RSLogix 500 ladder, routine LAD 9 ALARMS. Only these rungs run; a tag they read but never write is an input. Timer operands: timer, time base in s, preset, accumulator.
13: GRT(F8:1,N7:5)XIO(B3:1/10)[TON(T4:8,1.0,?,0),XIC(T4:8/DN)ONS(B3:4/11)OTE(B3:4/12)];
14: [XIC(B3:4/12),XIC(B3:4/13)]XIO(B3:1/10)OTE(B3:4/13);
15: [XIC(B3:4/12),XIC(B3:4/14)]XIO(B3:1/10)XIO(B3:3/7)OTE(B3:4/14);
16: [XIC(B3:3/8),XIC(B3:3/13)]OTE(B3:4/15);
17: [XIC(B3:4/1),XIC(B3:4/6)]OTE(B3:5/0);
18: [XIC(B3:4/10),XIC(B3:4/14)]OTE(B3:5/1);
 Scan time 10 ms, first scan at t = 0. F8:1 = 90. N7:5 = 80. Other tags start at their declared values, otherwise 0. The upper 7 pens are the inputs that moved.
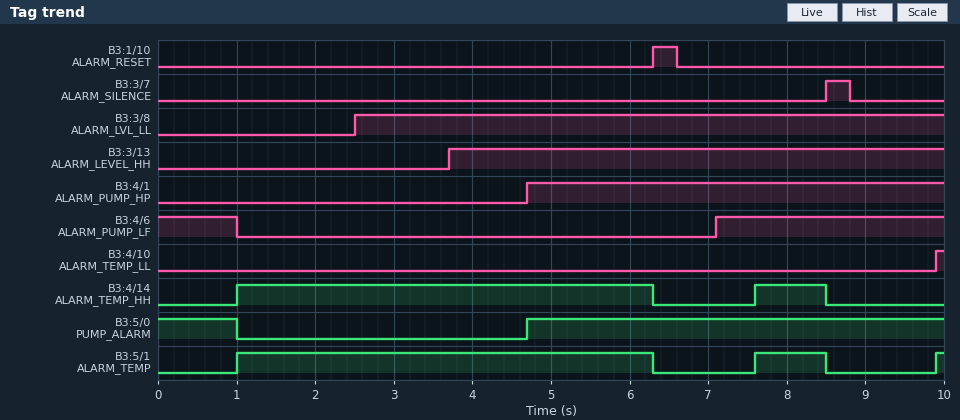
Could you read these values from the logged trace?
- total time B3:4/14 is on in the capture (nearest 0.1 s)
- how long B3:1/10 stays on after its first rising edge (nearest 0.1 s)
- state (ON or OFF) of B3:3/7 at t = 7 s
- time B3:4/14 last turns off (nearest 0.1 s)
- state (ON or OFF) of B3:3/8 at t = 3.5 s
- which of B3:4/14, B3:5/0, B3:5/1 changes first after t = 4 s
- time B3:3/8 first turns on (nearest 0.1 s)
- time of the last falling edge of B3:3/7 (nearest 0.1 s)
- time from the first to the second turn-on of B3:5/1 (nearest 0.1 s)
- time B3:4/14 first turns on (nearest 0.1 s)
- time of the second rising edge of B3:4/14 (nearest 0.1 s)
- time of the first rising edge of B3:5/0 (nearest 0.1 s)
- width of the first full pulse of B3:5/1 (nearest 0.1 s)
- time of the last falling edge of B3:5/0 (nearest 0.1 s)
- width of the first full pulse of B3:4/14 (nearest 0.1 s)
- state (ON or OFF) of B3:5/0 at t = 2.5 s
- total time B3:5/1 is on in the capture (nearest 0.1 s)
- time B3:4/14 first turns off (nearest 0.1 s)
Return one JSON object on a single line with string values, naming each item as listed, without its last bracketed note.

{"total time B3:4/14 is on in the capture": "6.2 s", "how long B3:1/10 stays on after its first rising edge": "0.3 s", "state (ON or OFF) of B3:3/7 at t = 7 s": "OFF", "time B3:4/14 last turns off": "8.5 s", "state (ON or OFF) of B3:3/8 at t = 3.5 s": "ON", "which of B3:4/14, B3:5/0, B3:5/1 changes first after t = 4 s": "B3:5/0", "time B3:3/8 first turns on": "2.5 s", "time of the last falling edge of B3:3/7": "8.8 s", "time from the first to the second turn-on of B3:5/1": "6.6 s", "time B3:4/14 first turns on": "1.0 s", "time of the second rising edge of B3:4/14": "7.6 s", "time of the first rising edge of B3:5/0": "4.7 s", "width of the first full pulse of B3:5/1": "5.3 s", "time of the last falling edge of B3:5/0": "1.0 s", "width of the first full pulse of B3:4/14": "5.3 s", "state (ON or OFF) of B3:5/0 at t = 2.5 s": "OFF", "total time B3:5/1 is on in the capture": "6.3 s", "time B3:4/14 first turns off": "6.3 s"}
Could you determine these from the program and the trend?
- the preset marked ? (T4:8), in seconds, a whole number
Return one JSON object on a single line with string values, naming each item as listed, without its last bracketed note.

{"the preset marked ? (T4:8), in seconds, a whole number": "1 s"}
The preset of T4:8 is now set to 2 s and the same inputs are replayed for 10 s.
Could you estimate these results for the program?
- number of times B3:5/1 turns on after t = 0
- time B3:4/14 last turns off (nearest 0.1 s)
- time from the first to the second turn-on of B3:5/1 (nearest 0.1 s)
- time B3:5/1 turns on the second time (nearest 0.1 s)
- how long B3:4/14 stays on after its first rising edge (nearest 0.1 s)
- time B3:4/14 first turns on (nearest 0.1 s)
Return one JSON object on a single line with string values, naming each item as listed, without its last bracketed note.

{"number of times B3:5/1 turns on after t = 0": "2", "time B3:4/14 last turns off": "6.3 s", "time from the first to the second turn-on of B3:5/1": "7.9 s", "time B3:5/1 turns on the second time": "9.9 s", "how long B3:4/14 stays on after its first rising edge": "4.3 s", "time B3:4/14 first turns on": "2.0 s"}
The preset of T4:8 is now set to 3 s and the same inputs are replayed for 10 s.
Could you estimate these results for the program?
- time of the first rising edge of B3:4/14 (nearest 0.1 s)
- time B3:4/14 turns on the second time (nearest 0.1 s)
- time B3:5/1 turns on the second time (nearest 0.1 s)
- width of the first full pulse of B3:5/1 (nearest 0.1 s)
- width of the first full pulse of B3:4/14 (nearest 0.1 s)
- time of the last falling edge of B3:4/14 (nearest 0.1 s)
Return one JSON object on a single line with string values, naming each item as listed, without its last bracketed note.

{"time of the first rising edge of B3:4/14": "3.0 s", "time B3:4/14 turns on the second time": "9.6 s", "time B3:5/1 turns on the second time": "9.6 s", "width of the first full pulse of B3:5/1": "3.3 s", "width of the first full pulse of B3:4/14": "3.3 s", "time of the last falling edge of B3:4/14": "6.3 s"}
